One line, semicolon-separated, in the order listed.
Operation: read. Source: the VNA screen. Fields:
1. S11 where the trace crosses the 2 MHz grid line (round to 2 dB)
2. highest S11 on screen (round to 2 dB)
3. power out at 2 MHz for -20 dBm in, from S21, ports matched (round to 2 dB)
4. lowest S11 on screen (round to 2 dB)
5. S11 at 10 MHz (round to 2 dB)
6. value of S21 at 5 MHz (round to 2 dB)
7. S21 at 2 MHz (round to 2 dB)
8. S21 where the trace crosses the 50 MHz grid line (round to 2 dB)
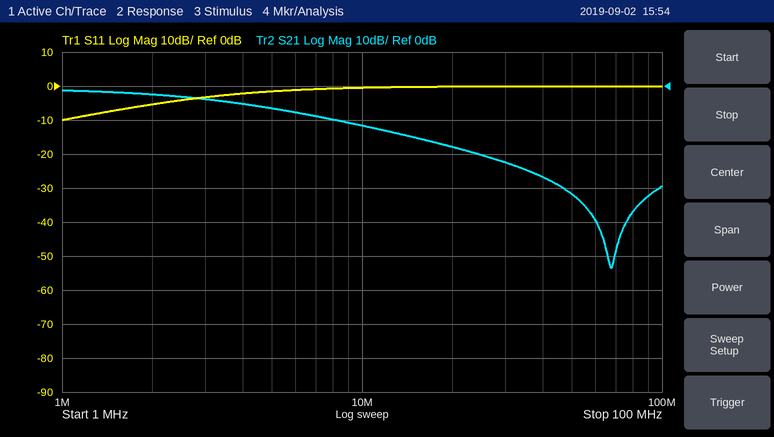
-6 dB; 0 dB; -22 dBm; -10 dB; 0 dB; -6 dB; -2 dB; -32 dB
